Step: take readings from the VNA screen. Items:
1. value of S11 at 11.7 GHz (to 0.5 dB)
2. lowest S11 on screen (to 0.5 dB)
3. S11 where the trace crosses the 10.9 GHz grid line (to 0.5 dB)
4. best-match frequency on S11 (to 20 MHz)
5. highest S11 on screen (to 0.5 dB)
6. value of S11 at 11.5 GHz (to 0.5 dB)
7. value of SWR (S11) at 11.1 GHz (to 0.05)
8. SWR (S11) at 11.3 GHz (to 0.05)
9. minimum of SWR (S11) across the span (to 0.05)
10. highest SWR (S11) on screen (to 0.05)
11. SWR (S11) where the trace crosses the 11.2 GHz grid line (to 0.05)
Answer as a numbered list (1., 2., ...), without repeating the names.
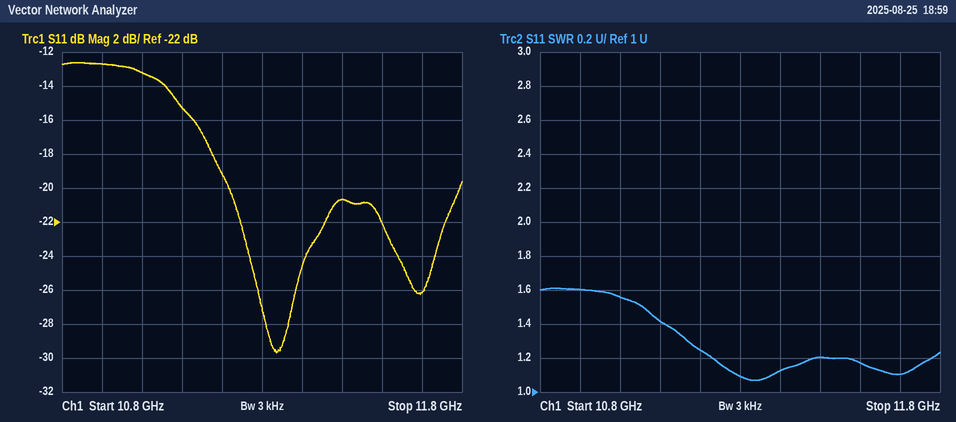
1. -26.0 dB
2. -29.5 dB
3. -12.5 dB
4. 11.34 GHz
5. -12.5 dB
6. -20.5 dB
7. 1.40
8. 1.10
9. 1.05
10. 1.60
11. 1.25
